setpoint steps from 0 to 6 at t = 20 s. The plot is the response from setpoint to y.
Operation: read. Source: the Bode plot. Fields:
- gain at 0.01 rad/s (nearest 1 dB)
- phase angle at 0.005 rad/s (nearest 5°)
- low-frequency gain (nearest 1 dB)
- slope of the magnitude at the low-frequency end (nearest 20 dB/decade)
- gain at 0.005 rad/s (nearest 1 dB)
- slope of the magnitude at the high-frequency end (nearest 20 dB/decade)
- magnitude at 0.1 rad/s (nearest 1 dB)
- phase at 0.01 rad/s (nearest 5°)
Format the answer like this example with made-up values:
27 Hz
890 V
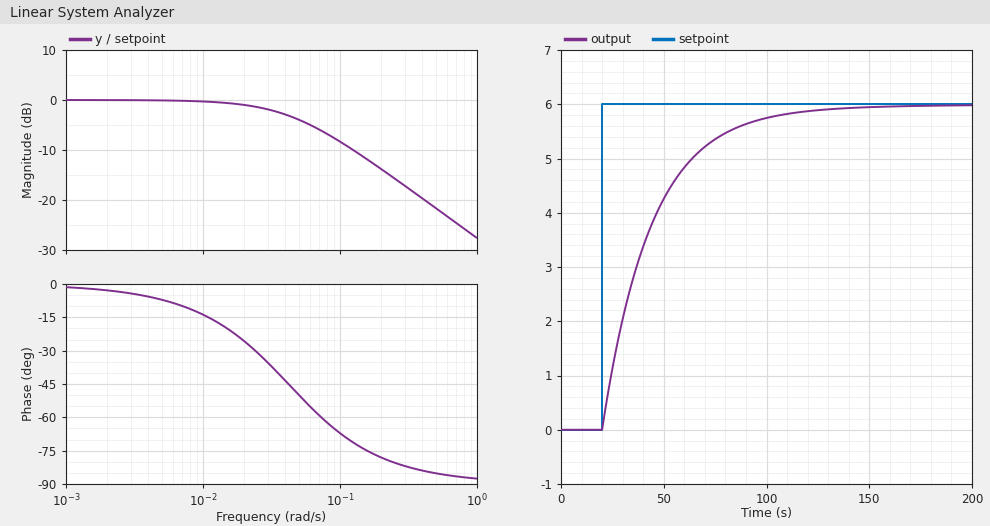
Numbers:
0 dB
-5°
0 dB
0 dB/decade
0 dB
-20 dB/decade
-8 dB
-15°
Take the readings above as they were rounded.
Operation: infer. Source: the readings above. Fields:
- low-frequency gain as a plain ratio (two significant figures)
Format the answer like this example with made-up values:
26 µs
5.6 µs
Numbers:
1.0
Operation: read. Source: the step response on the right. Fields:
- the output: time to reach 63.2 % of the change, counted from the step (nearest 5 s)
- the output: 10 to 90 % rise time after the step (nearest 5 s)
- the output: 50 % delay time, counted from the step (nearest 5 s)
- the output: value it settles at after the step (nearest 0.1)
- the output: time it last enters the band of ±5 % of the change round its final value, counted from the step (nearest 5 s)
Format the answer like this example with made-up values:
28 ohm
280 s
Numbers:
25 s
55 s
15 s
6.0
75 s
